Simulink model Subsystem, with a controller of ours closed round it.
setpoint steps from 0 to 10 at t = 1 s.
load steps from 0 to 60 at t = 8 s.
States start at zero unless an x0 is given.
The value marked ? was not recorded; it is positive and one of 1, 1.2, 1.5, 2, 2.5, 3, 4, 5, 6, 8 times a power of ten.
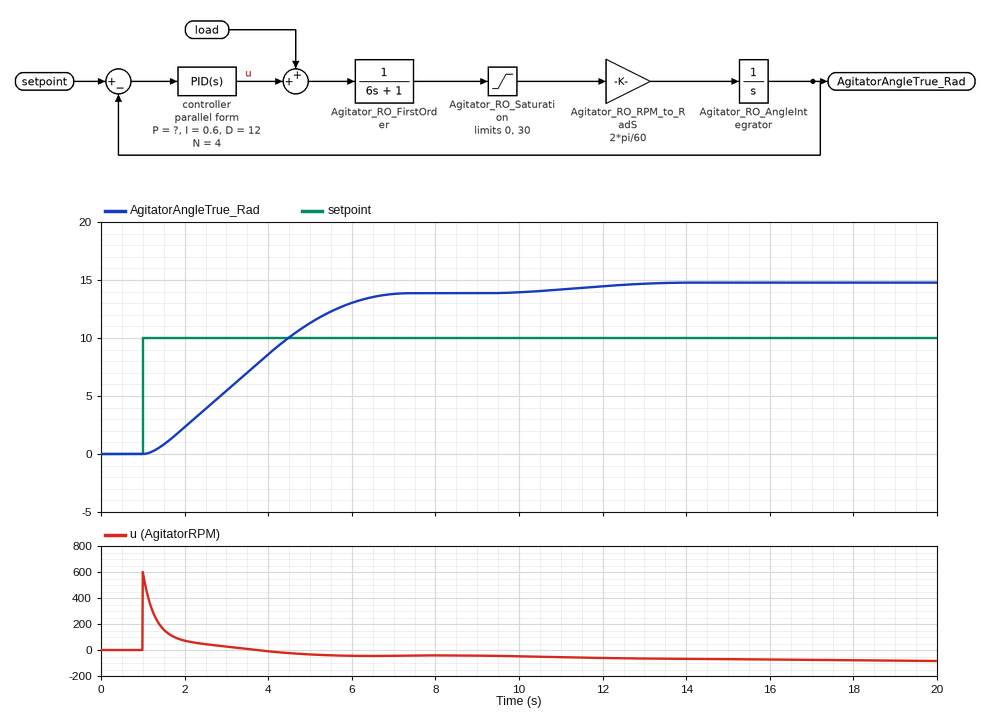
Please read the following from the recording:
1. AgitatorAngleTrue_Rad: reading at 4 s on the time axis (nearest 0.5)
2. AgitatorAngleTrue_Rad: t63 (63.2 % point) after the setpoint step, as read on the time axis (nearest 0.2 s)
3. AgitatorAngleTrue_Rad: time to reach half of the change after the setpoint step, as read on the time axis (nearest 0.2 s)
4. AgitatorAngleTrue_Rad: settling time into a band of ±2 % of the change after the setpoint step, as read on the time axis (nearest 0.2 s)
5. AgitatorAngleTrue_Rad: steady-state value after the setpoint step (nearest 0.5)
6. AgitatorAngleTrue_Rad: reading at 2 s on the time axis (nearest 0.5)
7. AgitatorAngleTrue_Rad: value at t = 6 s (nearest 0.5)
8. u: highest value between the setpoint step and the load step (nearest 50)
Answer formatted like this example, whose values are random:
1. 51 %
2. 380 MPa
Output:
1. 8.5
2. 4.0 s
3. 3.4 s
4. 6.6 s
5. 14.0
6. 2.5
7. 13.0
8. 600
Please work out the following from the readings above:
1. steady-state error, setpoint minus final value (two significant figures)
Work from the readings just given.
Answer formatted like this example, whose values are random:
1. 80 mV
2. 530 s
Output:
1. -4.0
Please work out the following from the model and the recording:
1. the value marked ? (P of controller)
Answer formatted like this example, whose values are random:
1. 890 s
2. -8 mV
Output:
1. 12
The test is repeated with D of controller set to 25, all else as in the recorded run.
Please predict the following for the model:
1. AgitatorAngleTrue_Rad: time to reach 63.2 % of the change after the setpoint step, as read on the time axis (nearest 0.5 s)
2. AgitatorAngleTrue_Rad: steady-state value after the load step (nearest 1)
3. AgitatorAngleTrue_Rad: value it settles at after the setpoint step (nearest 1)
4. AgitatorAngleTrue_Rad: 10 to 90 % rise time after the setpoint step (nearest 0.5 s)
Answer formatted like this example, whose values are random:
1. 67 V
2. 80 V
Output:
1. 3.5 s
2. 15
3. 12
4. 3.5 s
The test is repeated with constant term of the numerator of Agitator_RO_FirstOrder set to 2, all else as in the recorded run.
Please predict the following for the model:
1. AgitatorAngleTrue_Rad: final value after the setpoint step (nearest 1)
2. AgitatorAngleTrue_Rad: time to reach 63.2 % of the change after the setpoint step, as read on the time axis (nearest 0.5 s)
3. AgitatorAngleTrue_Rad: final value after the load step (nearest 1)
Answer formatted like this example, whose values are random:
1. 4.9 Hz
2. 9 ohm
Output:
1. 15
2. 4.0 s
3. 15
